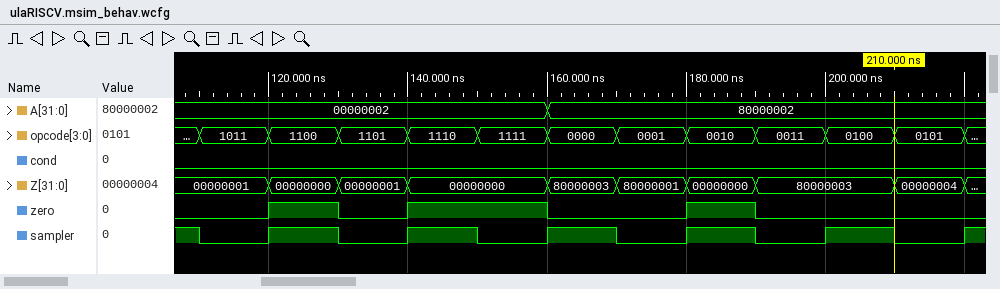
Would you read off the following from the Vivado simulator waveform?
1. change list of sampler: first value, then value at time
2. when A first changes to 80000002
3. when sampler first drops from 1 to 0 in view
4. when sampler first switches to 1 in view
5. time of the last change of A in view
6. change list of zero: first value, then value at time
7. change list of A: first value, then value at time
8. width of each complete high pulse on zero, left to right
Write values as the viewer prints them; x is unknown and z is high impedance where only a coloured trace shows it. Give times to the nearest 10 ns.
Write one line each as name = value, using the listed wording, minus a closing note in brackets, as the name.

change list of sampler: first value, then value at time = 1, 0 at 110 ns, 1 at 120 ns, 0 at 130 ns, 1 at 140 ns, 0 at 150 ns, 1 at 160 ns, 0 at 170 ns, 1 at 180 ns, 0 at 190 ns, 1 at 200 ns, 0 at 210 ns, 1 at 220 ns
when A first changes to 80000002 = 160 ns
when sampler first drops from 1 to 0 in view = 110 ns
when sampler first switches to 1 in view = 120 ns
time of the last change of A in view = 160 ns
change list of zero: first value, then value at time = 0, 1 at 120 ns, 0 at 130 ns, 1 at 140 ns, 0 at 160 ns, 1 at 180 ns, 0 at 190 ns
change list of A: first value, then value at time = 00000002, 80000002 at 160 ns
width of each complete high pulse on zero, left to right = 10 ns, 20 ns, 10 ns
